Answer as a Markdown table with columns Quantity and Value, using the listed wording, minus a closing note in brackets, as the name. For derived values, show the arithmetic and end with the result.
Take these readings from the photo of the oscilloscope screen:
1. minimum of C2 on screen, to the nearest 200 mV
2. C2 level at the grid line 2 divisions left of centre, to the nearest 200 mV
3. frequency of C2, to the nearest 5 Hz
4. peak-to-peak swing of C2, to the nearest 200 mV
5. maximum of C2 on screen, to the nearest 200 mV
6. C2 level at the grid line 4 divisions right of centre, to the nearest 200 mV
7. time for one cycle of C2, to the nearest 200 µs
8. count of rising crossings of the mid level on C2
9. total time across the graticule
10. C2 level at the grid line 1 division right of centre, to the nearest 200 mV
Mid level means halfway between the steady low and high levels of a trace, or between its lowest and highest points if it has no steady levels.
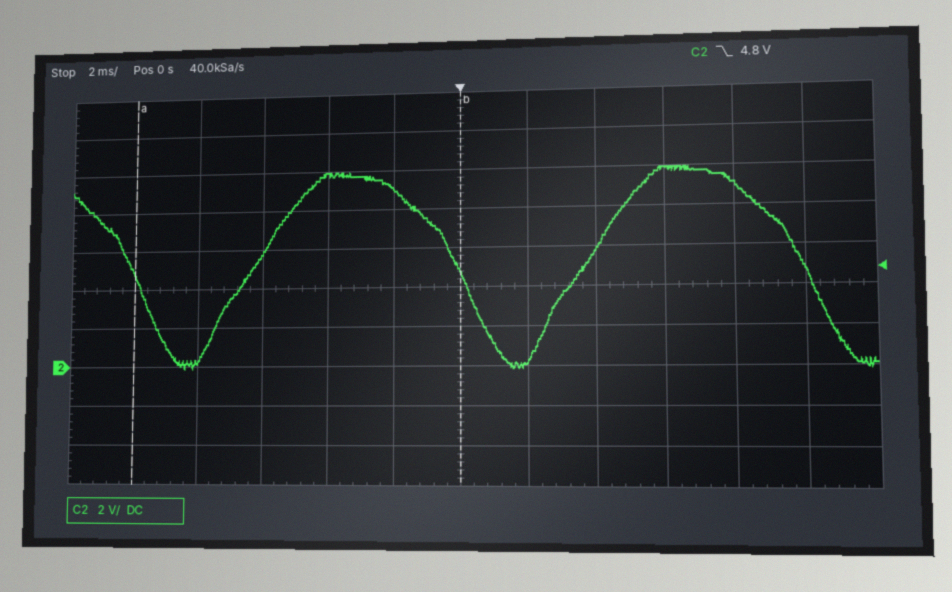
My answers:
| Quantity | Value |
|---|---|
| minimum of C2 on screen, to the nearest 200 mV | 0.0 V |
| C2 level at the grid line 2 divisions left of centre, to the nearest 200 mV | 9.8 V |
| frequency of C2, to the nearest 5 Hz | 1 / 10.0 ms ≈ 100 Hz |
| peak-to-peak swing of C2, to the nearest 200 mV | 10.0 V − (0.0 V) = 10.0 V |
| maximum of C2 on screen, to the nearest 200 mV | 10.0 V |
| C2 level at the grid line 4 divisions right of centre, to the nearest 200 mV | 9.0 V |
| time for one cycle of C2, to the nearest 200 µs | 10.0 ms |
| count of rising crossings of the mid level on C2 | 2 |
| total time across the graticule | 24 ms |
| C2 level at the grid line 1 division right of centre, to the nearest 200 mV | 200 mV |
